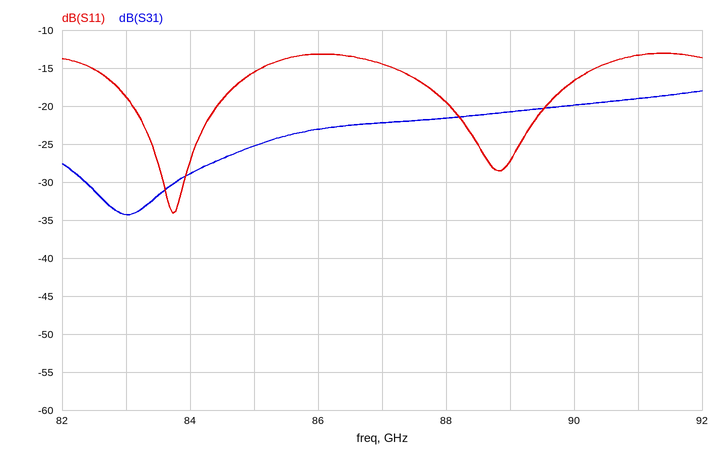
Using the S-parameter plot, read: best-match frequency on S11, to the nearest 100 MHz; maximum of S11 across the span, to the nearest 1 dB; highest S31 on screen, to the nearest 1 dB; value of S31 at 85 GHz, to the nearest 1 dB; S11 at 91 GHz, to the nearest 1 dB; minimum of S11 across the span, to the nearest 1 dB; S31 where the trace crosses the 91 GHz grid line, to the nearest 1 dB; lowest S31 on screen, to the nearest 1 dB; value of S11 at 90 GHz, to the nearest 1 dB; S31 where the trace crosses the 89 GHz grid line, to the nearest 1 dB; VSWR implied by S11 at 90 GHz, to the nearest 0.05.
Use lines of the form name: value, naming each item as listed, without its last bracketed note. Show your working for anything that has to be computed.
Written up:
best-match frequency on S11, to the nearest 100 MHz: 83.7 GHz
maximum of S11 across the span, to the nearest 1 dB: -13 dB
highest S31 on screen, to the nearest 1 dB: -18 dB
value of S31 at 85 GHz, to the nearest 1 dB: -25 dB
S11 at 91 GHz, to the nearest 1 dB: -13 dB
minimum of S11 across the span, to the nearest 1 dB: -34 dB
S31 where the trace crosses the 91 GHz grid line, to the nearest 1 dB: -19 dB
lowest S31 on screen, to the nearest 1 dB: -34 dB
value of S11 at 90 GHz, to the nearest 1 dB: -17 dB
S31 where the trace crosses the 89 GHz grid line, to the nearest 1 dB: -21 dB
VSWR implied by S11 at 90 GHz, to the nearest 0.05: |Γ| = 10^(-17/20) = 0.1413; VSWR = (1 + 0.1413)/(1 − 0.1413) ≈ 1.33, so 1.35 to the nearest 0.05
